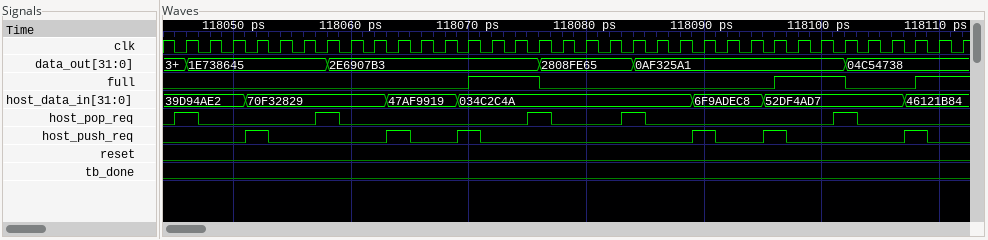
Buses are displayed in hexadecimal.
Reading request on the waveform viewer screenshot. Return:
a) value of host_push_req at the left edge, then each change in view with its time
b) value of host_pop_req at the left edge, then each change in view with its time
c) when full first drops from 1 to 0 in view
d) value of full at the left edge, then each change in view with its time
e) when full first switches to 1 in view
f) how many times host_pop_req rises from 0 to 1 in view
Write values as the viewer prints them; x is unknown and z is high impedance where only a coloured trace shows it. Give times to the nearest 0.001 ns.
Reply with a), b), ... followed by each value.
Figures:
a) 0, 1 at 118.051 ns, 0 at 118.053 ns, 1 at 118.063 ns, 0 at 118.065 ns, 1 at 118.069 ns, 0 at 118.071 ns, 1 at 118.089 ns, 0 at 118.091 ns, 1 at 118.095 ns, 0 at 118.097 ns, 1 at 118.107 ns, 0 at 118.109 ns
b) 0, 1 at 118.045 ns, 0 at 118.047 ns, 1 at 118.057 ns, 0 at 118.059 ns, 1 at 118.075 ns, 0 at 118.077 ns, 1 at 118.083 ns, 0 at 118.085 ns, 1 at 118.101 ns, 0 at 118.103 ns
c) 118.076 ns
d) 0, 1 at 118.07 ns, 0 at 118.076 ns, 1 at 118.096 ns, 0 at 118.102 ns, 1 at 118.108 ns
e) 118.07 ns
f) 5
